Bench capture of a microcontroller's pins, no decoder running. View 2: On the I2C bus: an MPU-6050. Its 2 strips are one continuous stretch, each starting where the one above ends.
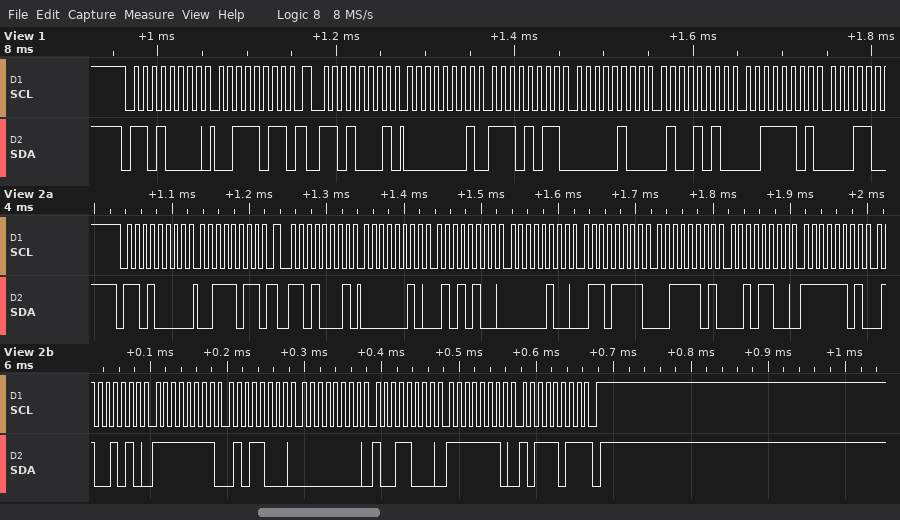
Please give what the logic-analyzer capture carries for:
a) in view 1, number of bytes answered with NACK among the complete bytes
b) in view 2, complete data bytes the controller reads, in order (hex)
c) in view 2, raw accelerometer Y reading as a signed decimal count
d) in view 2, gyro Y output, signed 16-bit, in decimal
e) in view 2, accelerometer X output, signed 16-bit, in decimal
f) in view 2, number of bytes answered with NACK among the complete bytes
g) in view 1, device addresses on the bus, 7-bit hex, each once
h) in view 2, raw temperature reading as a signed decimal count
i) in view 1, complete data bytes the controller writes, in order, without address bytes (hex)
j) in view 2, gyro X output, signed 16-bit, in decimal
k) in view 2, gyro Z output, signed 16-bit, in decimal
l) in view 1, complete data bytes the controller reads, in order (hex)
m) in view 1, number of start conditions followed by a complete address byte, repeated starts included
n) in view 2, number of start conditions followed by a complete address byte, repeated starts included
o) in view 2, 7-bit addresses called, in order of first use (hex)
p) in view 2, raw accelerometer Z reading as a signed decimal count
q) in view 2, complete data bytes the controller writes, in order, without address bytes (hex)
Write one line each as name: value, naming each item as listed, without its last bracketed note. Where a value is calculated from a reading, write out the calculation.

in view 1, number of bytes answered with NACK among the complete bytes: 0
in view 2, complete data bytes the controller reads, in order: 02 54 04 6F 3D 2C FD 4A FF 58 00 98 FE BB
in view 2, raw accelerometer Y reading as a signed decimal count: 0x046F = 1135
in view 2, gyro Y output, signed 16-bit, in decimal: 0x0098 = 152
in view 2, accelerometer X output, signed 16-bit, in decimal: 0x0254 = 596
in view 2, number of bytes answered with NACK among the complete bytes: 1
in view 1, device addresses on the bus, 7-bit hex, each once: 0x68
in view 2, raw temperature reading as a signed decimal count: 0xFD4A = -694
in view 1, complete data bytes the controller writes, in order, without address bytes: 3B
in view 2, gyro X output, signed 16-bit, in decimal: 0xFF58 = -168
in view 2, gyro Z output, signed 16-bit, in decimal: 0xFEBB = -325
in view 1, complete data bytes the controller reads, in order: 01 EB 04 4A 3D
in view 1, number of start conditions followed by a complete address byte, repeated starts included: 2
in view 2, number of start conditions followed by a complete address byte, repeated starts included: 2
in view 2, 7-bit addresses called, in order of first use: 0x68
in view 2, raw accelerometer Z reading as a signed decimal count: 0x3D2C = 15660
in view 2, complete data bytes the controller writes, in order, without address bytes: 3B
